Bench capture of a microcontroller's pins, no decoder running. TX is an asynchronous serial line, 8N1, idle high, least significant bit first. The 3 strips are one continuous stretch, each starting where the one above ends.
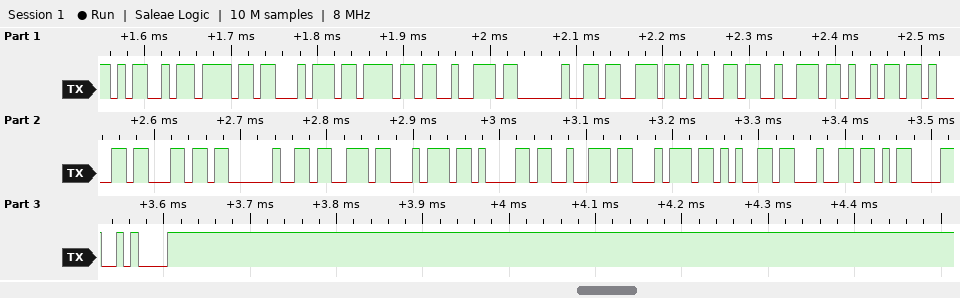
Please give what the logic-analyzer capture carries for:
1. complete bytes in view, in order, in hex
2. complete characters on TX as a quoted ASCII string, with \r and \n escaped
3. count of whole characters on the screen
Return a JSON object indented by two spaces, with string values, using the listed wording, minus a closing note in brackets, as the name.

{
  "complete bytes in view, in order, in hex": "0x4D 0x6F 0x74 0x6F 0x72 0x20 0x73 0x65 0x72 0x69 0x61 0x6C 0x20 0x73 0x74 0x61 0x72 0x74 0x65 0x64 0x0D 0x0A",
  "complete characters on TX as a quoted ASCII string, with \\r and \\n escaped": "\"Motor serial started\\r\\n\"",
  "count of whole characters on the screen": "22"
}
